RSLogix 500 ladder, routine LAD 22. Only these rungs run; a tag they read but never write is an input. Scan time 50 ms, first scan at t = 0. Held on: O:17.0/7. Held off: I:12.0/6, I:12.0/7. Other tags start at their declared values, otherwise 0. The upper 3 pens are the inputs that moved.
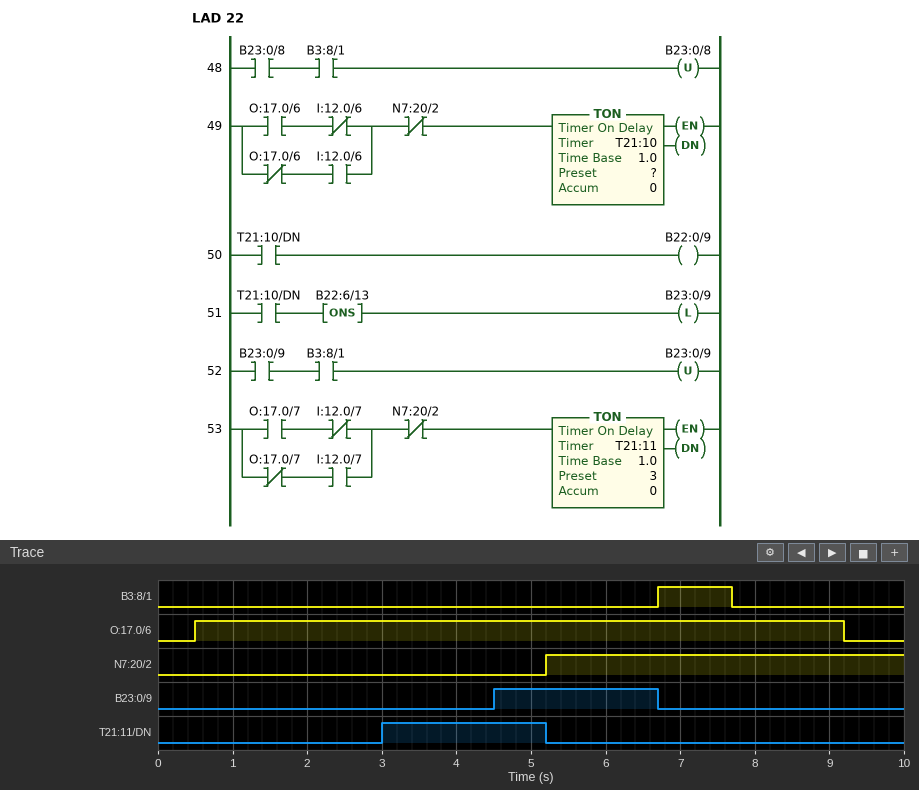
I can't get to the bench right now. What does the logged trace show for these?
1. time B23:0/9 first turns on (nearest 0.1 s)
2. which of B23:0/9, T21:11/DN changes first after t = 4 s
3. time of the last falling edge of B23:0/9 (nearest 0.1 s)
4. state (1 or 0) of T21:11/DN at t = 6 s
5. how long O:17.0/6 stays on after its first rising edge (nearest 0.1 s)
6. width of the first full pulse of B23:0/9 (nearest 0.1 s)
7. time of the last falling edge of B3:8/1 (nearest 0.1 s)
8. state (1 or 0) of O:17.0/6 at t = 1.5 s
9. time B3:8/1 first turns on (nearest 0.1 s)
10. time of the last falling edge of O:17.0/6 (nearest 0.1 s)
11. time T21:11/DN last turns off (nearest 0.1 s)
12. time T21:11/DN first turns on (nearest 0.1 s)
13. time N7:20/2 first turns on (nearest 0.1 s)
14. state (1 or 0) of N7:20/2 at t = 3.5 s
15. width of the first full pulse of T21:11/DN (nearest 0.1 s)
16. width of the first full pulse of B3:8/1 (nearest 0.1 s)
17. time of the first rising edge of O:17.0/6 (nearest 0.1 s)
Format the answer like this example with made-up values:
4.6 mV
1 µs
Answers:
4.5 s
B23:0/9
6.7 s
0
8.7 s
2.2 s
7.7 s
1
6.7 s
9.2 s
5.2 s
3.0 s
5.2 s
0
2.2 s
1.0 s
0.5 s
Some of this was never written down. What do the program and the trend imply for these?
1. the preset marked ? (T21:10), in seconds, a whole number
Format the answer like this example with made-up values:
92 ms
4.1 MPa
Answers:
4 s
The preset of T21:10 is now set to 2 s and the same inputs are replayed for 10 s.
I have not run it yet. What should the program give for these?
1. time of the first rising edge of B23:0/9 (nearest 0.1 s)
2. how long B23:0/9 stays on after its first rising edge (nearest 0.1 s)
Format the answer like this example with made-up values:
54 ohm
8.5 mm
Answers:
2.5 s
4.2 s
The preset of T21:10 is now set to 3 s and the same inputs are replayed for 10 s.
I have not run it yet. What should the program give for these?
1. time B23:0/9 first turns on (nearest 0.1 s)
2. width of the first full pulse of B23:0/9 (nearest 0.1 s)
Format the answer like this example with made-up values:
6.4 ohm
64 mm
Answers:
3.5 s
3.2 s
